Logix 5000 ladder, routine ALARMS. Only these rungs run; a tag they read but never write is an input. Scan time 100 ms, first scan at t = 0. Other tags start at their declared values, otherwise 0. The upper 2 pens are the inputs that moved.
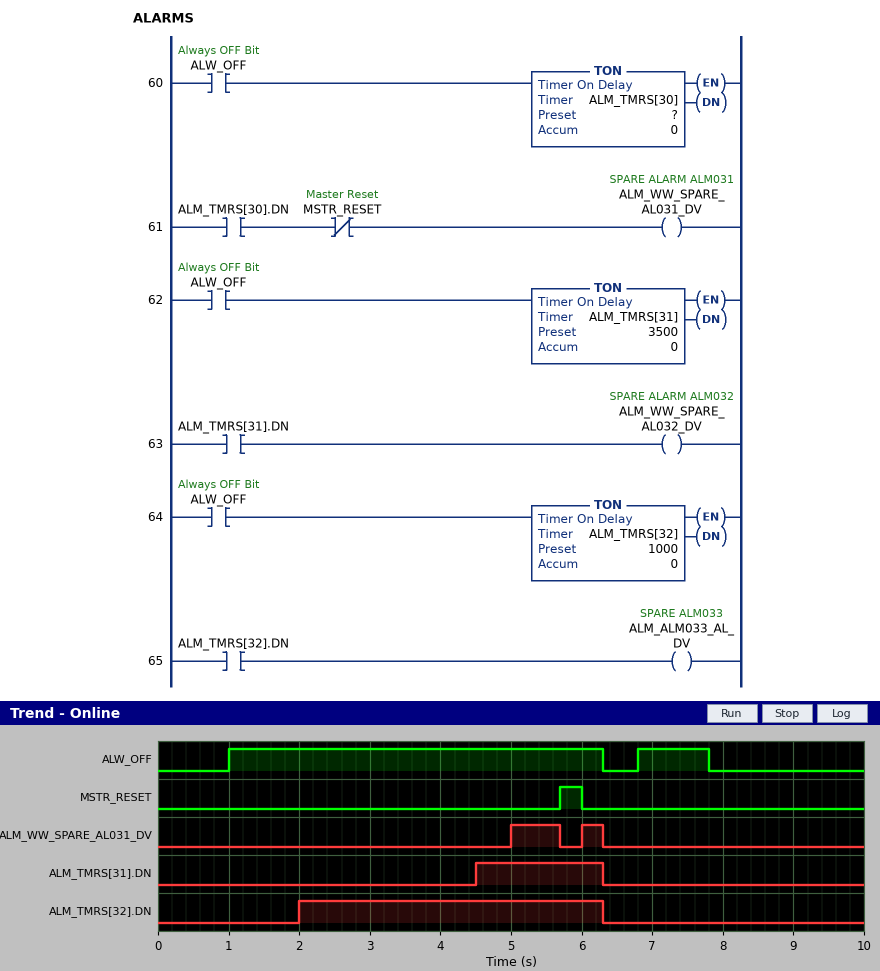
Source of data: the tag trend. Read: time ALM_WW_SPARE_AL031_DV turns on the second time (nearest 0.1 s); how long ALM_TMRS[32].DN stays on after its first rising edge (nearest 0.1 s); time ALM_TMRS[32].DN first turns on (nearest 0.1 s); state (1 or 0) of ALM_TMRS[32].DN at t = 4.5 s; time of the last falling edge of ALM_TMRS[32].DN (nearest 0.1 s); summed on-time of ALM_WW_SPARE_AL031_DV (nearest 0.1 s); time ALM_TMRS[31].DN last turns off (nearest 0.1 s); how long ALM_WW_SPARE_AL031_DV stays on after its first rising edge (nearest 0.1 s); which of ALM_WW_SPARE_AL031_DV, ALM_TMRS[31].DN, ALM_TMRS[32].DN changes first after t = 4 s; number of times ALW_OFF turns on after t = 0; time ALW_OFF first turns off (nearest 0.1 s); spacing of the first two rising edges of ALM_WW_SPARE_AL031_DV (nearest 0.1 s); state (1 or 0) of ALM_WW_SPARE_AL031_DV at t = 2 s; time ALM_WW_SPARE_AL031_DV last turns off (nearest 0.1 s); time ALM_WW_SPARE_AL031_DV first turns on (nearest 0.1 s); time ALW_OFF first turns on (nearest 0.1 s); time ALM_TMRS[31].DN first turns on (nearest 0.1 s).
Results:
6.0 s
4.3 s
2.0 s
1
6.3 s
1.0 s
6.3 s
0.7 s
ALM_TMRS[31].DN
2
6.3 s
1.0 s
0
6.3 s
5.0 s
1.0 s
4.5 s
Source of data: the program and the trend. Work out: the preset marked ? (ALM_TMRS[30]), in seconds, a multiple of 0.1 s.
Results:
4.0 s
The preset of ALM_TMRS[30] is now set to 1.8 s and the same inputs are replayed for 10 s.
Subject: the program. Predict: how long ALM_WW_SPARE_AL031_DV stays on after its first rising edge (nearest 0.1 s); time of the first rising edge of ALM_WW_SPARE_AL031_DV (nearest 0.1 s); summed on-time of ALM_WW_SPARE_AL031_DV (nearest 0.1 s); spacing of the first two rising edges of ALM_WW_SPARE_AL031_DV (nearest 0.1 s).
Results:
2.9 s
2.8 s
3.2 s
3.2 s
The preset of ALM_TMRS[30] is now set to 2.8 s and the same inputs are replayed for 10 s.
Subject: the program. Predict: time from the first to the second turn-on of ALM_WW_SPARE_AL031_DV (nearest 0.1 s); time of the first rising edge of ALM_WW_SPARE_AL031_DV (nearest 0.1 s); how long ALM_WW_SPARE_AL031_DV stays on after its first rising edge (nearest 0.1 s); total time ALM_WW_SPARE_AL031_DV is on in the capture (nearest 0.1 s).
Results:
2.2 s
3.8 s
1.9 s
2.2 s
